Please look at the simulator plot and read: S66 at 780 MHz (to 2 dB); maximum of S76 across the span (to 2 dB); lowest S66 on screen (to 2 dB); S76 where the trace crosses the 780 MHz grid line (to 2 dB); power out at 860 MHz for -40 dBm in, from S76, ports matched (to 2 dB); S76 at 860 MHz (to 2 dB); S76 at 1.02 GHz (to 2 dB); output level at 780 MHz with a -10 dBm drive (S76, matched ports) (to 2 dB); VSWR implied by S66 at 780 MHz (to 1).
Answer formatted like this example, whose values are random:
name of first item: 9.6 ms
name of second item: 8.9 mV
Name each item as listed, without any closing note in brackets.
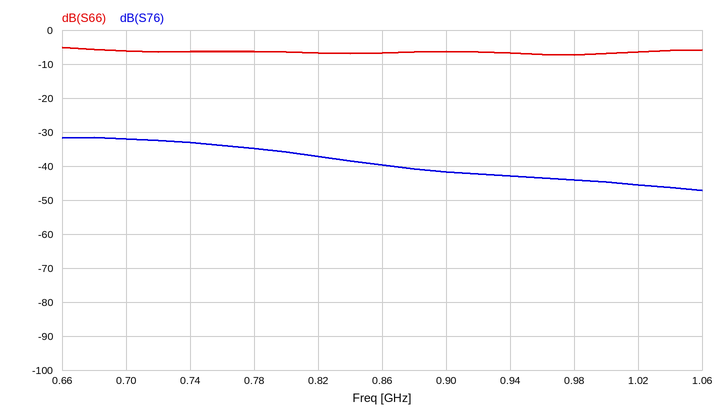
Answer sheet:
S66 at 780 MHz: -6 dB
maximum of S76 across the span: -32 dB
lowest S66 on screen: -8 dB
S76 where the trace crosses the 780 MHz grid line: -34 dB
power out at 860 MHz for -40 dBm in, from S76, ports matched: -80 dBm
S76 at 860 MHz: -40 dB
S76 at 1.02 GHz: -46 dB
output level at 780 MHz with a -10 dBm drive (S76, matched ports): -44 dBm
VSWR implied by S66 at 780 MHz: 3
